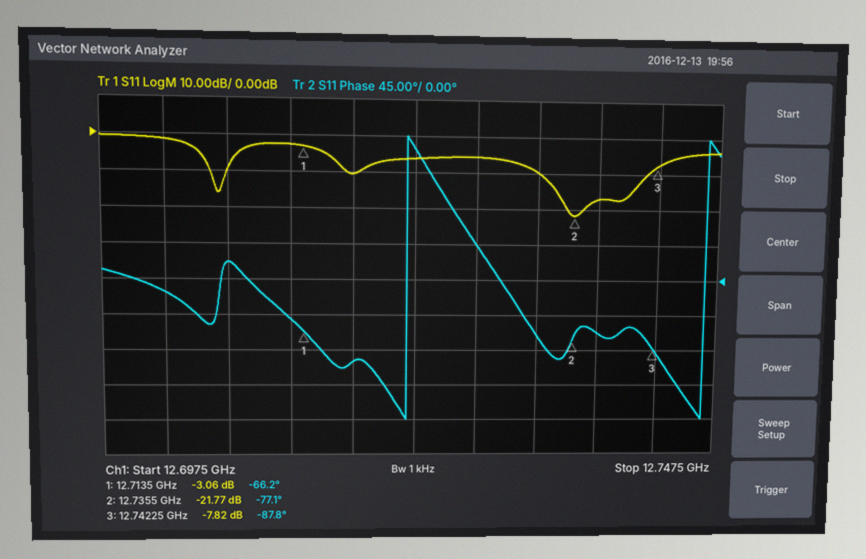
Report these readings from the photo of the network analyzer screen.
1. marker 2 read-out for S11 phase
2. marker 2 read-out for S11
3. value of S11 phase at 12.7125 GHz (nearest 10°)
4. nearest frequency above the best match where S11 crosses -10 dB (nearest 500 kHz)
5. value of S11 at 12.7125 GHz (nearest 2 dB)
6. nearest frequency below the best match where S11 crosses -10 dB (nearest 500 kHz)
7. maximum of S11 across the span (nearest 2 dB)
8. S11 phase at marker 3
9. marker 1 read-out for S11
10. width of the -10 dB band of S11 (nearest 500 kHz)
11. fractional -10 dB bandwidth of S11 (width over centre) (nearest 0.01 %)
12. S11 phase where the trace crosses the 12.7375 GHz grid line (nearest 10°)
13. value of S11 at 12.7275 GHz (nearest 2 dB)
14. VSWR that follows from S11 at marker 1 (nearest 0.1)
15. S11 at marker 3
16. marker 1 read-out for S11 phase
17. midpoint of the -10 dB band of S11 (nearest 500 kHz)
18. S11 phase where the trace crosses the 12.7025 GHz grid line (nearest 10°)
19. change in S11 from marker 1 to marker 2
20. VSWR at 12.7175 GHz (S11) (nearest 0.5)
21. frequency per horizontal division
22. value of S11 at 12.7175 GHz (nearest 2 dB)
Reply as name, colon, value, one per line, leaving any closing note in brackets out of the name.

marker 2 read-out for S11 phase: -77.1°
marker 2 read-out for S11: -21.77 dB
value of S11 phase at 12.7125 GHz: -50°
nearest frequency above the best match where S11 crosses -10 dB: 12.7415 GHz
value of S11 at 12.7125 GHz: -2 dB
nearest frequency below the best match where S11 crosses -10 dB: 12.7325 GHz
maximum of S11 across the span: 0 dB
S11 phase at marker 3: -87.8°
marker 1 read-out for S11: -3.06 dB
width of the -10 dB band of S11: 9.0 MHz
fractional -10 dB bandwidth of S11 (width over centre): 0.07 %
S11 phase where the trace crosses the 12.7375 GHz grid line: -70°
value of S11 at 12.7275 GHz: -6 dB
VSWR that follows from S11 at marker 1: 5.7
S11 at marker 3: -7.82 dB
marker 1 read-out for S11 phase: -66.2°
midpoint of the -10 dB band of S11: 12.7370 GHz
S11 phase where the trace crosses the 12.7025 GHz grid line: -20°
change in S11 from marker 1 to marker 2: -18.71 dB
VSWR at 12.7175 GHz (S11): 2.0
frequency per horizontal division: 5 MHz
value of S11 at 12.7175 GHz: -10 dB
